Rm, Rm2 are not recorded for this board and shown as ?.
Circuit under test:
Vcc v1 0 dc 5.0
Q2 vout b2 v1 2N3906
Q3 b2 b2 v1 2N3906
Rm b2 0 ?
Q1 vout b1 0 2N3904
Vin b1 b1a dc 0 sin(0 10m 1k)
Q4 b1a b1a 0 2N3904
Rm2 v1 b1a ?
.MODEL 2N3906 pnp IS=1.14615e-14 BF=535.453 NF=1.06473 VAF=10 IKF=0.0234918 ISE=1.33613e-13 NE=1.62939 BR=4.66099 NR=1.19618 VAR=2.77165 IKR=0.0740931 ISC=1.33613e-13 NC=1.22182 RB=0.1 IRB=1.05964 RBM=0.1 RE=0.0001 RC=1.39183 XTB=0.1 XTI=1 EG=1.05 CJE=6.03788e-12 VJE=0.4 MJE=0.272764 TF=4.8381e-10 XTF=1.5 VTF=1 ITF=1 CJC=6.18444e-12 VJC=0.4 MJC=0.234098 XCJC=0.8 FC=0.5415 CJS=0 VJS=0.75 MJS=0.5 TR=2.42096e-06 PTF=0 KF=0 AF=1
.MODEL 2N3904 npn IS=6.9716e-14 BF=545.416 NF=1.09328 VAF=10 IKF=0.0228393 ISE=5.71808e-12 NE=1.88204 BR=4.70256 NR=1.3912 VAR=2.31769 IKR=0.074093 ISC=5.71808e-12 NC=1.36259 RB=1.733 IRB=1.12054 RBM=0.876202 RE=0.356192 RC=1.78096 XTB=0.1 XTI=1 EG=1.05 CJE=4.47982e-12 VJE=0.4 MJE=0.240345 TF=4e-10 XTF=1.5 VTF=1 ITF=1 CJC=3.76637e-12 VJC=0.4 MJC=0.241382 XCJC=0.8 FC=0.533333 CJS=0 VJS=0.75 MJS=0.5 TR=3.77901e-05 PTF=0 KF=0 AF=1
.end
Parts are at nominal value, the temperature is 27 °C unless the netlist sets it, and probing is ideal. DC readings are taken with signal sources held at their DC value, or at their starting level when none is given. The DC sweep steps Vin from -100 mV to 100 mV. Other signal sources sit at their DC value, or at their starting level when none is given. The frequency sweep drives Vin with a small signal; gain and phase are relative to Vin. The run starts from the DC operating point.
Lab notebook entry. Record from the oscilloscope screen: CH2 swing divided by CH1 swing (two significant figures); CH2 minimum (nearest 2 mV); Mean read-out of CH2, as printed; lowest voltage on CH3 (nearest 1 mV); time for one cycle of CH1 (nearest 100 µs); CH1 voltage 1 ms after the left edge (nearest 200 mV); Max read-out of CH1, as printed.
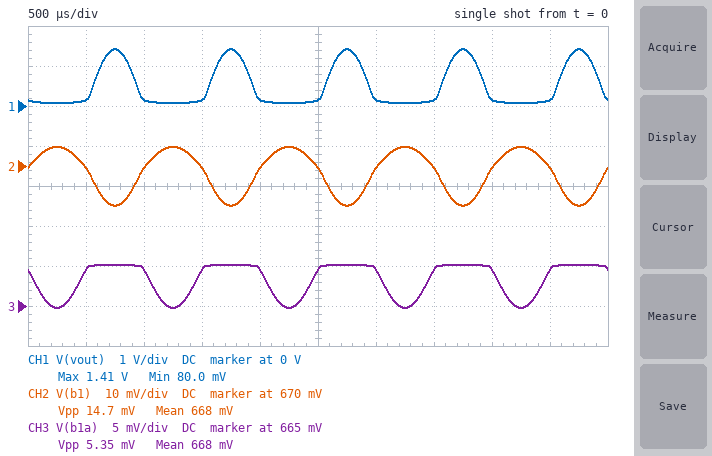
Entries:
0.011
660 mV
668 mV
665 mV
1.0 ms
200 mV
1.41 V
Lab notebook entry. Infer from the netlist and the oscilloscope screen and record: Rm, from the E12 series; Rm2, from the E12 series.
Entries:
8.2 kΩ
4.7 kΩ
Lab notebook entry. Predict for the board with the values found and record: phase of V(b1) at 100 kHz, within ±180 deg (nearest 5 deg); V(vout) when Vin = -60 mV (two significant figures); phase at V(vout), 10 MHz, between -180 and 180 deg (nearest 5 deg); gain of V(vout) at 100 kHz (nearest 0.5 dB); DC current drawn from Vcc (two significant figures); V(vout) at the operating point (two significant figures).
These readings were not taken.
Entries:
0 deg
5.0 V
70 deg
27.5 dB
2.3 mA
150 mV
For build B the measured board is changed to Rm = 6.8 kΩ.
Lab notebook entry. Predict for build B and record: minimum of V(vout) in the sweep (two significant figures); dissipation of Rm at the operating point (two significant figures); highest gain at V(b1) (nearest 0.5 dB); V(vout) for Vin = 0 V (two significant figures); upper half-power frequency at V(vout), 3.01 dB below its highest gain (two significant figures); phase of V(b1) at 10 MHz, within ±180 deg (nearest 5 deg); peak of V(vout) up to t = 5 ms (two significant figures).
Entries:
34 mV
2.7 mW
0 dB
790 mV
2.1 MHz
-5 deg
2.3 V
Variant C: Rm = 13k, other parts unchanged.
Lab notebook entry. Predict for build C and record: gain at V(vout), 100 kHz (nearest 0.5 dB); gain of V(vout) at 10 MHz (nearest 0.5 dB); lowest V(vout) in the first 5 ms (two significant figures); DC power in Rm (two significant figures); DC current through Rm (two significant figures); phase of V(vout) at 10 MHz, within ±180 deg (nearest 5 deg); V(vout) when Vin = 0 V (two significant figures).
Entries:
5.5 dB
-5.5 dB
46 mV
1.4 mW
330 µA
15 deg
60 mV
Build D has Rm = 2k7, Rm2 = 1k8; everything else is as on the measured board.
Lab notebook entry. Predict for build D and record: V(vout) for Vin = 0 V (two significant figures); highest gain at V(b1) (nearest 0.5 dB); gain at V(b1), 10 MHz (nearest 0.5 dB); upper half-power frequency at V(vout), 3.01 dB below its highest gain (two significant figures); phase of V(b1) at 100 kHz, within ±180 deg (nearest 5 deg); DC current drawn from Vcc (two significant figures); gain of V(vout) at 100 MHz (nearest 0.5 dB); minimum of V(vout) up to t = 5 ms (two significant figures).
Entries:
660 mV
0 dB
-1.5 dB
5.0 MHz
0 deg
6.3 mA
17.0 dB
100 mV
